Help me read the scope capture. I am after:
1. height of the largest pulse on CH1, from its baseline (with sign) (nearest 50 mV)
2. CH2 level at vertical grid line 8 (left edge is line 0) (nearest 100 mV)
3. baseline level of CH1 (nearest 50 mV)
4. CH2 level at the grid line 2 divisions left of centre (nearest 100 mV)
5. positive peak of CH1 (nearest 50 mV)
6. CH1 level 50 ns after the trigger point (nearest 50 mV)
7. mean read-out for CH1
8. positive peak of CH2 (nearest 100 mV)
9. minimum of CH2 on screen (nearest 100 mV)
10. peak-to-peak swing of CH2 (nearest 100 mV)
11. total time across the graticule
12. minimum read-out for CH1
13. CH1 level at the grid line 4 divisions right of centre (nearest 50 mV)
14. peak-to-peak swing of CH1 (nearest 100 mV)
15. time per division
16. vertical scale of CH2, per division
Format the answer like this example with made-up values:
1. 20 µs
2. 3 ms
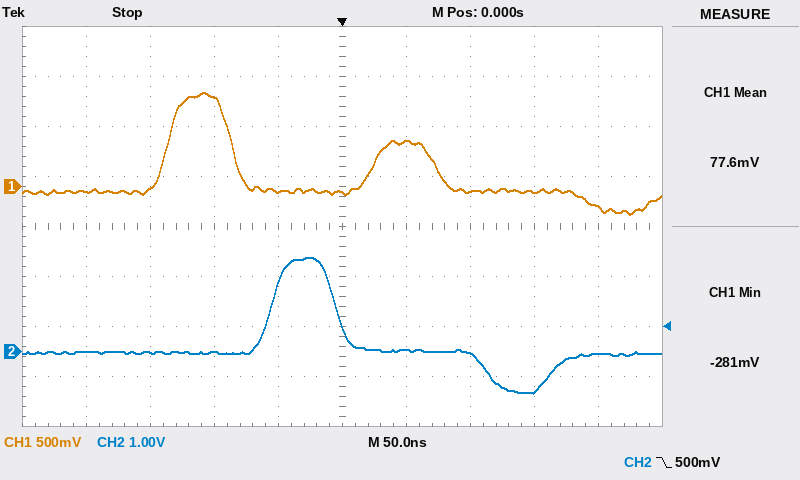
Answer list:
1. +1.00 V
2. -800 mV
3. -50 mV
4. 0.0 V
5. 950 mV
6. 450 mV
7. 77.6 mV
8. 1.9 V
9. -800 mV
10. 2.7 V
11. 500 ns
12. -281 mV
13. -200 mV
14. 1.20 V
15. 50 ns
16. 1 V
